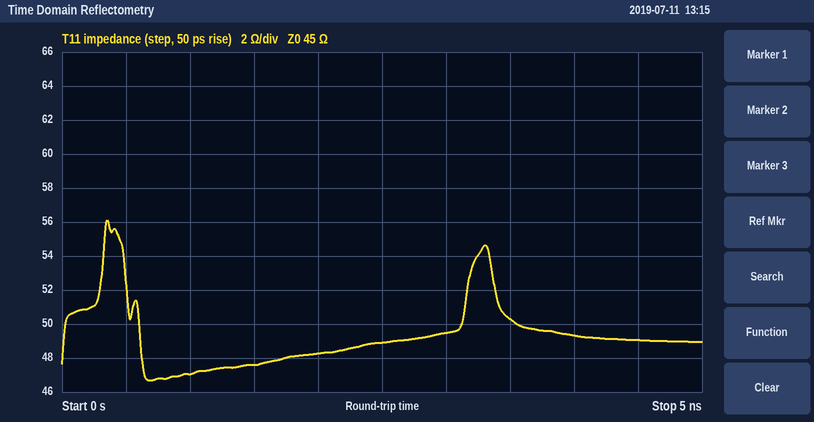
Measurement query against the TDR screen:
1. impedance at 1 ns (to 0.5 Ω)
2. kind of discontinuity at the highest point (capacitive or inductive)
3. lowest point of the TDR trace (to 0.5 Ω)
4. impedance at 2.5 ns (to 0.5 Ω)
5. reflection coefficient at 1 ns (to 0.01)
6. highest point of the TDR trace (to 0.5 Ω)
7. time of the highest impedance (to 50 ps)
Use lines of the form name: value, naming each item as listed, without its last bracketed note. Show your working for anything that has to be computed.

impedance at 1 ns: 47.0 Ω
kind of discontinuity at the highest point: inductive
lowest point of the TDR trace: 46.5 Ω
impedance at 2.5 ns: 49.0 Ω
reflection coefficient at 1 ns: (47 − 45)/(47 + 45) ≈ +0.02
highest point of the TDR trace: 56.0 Ω
time of the highest impedance: 350 ps
